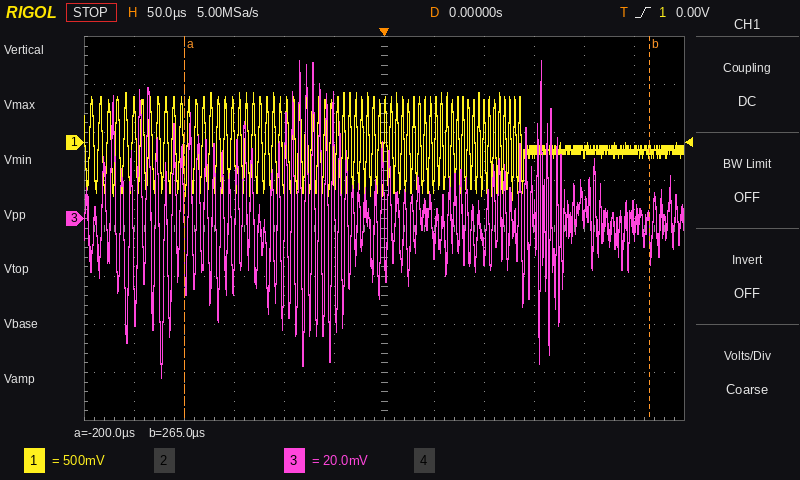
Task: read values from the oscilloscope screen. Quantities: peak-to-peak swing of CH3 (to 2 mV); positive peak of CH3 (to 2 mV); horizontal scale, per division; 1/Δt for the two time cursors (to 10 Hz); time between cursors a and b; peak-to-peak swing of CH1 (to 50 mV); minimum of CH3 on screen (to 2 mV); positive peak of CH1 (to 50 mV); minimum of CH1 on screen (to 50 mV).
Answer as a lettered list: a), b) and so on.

a) 132 mV
b) 66 mV
c) 50 µs
d) 2.15 kHz
e) 465 µs
f) 1.10 V
g) -66 mV
h) 500 mV
i) -600 mV
